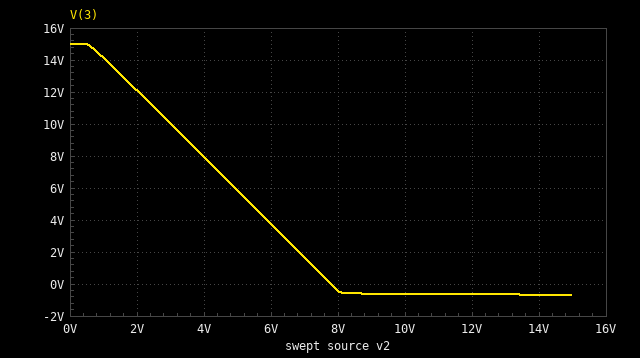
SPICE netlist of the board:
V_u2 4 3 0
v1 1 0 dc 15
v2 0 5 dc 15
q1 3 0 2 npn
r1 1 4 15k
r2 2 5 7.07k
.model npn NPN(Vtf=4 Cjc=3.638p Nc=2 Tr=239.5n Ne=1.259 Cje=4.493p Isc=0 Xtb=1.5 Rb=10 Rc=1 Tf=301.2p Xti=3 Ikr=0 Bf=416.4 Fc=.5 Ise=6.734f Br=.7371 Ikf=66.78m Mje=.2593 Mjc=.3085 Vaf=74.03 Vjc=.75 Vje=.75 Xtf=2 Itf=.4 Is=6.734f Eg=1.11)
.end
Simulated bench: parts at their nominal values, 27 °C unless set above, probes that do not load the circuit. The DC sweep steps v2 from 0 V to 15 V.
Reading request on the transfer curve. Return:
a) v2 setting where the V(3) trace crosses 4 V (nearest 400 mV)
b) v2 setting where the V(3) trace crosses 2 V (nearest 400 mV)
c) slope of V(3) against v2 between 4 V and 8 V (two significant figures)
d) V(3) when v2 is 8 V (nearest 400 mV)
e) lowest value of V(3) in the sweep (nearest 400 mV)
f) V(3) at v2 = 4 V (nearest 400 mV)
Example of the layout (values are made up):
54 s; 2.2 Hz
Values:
6.0 V; 6.8 V; -2.1 V/V; -400 mV; -800 mV; 8.0 V
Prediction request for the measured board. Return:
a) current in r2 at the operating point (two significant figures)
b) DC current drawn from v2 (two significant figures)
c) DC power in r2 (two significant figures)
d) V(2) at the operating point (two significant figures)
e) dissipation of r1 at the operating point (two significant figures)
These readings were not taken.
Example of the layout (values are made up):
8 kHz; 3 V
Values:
2.0 mA; 2.0 mA; 29 mW; -700 mV; 16 mW
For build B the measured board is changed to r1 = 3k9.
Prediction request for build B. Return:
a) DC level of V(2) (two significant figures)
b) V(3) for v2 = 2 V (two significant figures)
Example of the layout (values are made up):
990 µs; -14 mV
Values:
-680 mV; 14 V
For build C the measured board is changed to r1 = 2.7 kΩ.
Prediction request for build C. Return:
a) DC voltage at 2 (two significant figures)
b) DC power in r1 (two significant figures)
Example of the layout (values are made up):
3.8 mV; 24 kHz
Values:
-680 mV; 11 mW
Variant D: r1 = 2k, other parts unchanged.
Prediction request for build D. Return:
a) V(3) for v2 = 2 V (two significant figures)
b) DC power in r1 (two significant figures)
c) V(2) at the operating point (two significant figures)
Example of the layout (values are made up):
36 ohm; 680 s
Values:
15 V; 8.1 mW; -680 mV
